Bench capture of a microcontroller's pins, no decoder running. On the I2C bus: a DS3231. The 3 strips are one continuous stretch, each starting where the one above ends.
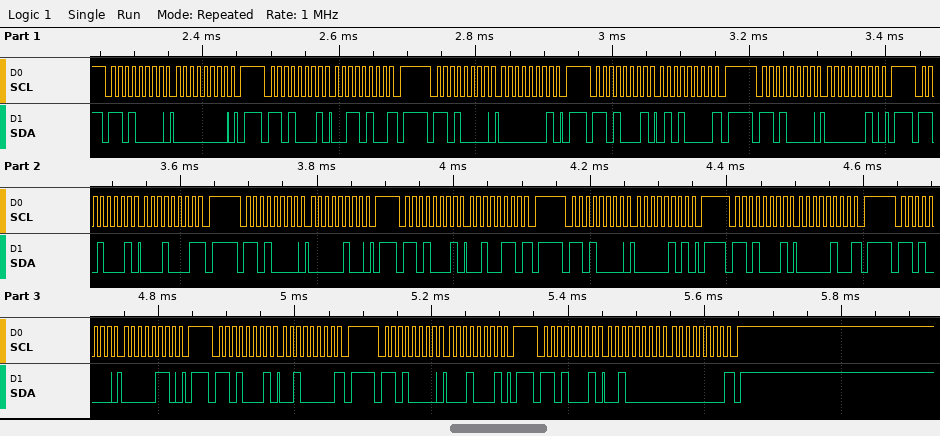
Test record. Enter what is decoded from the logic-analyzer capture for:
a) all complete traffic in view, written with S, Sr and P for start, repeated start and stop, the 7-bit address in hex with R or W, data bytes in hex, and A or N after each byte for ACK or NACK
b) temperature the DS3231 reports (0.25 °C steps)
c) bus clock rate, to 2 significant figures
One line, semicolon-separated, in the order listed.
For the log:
S 68W A 00 A P S 68R A 34 N P S 68W A 01 A P S 68R A 50 N P S 68W A 02 A P S 68R A 11 N P S 68W A 04 A P S 68R A 26 N P S 68W A 05 A P S 68R A 04 N P S 68W A 06 A P S 68R A 20 N P S 68W A 11 A P S 68R A 20 A 00 N P; 32.00 °C; 100 kHz
